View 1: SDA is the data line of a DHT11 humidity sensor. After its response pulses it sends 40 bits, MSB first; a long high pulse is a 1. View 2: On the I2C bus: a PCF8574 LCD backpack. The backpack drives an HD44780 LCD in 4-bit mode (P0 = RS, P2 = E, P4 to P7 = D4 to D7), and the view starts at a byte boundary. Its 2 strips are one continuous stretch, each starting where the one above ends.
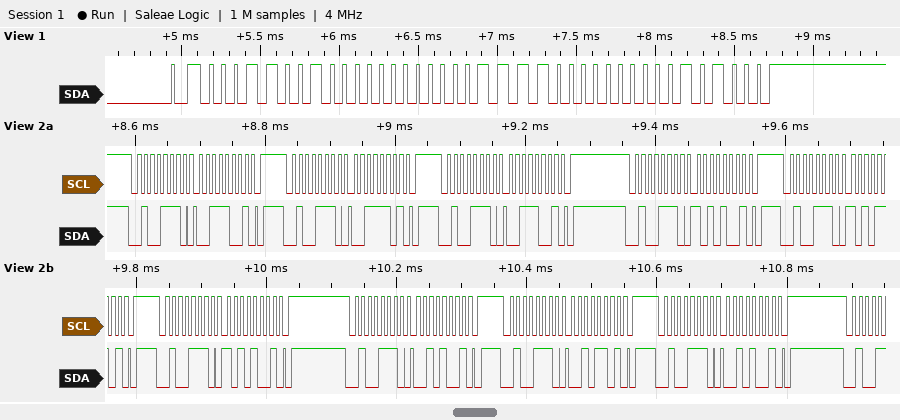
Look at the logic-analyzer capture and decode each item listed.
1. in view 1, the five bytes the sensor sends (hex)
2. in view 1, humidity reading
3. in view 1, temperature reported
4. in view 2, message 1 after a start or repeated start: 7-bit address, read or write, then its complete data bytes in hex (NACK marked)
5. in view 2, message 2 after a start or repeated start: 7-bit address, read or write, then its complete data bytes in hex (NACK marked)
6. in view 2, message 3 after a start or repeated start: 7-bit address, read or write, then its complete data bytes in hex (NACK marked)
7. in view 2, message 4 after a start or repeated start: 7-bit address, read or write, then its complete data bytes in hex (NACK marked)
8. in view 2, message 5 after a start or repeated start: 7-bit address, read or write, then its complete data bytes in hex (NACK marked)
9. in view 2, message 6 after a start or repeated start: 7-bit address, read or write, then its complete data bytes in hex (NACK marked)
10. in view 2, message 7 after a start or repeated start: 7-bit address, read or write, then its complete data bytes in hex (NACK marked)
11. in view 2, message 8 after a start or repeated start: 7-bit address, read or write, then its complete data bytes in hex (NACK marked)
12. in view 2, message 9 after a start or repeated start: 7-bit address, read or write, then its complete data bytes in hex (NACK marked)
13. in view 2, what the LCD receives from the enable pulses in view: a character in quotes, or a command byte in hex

19 00 0F 00 28
25 %
15.0 °C
0x27 write: 39
0x27 write: 3D
0x27 write: 39
0x27 write: A9
0x27 write: AD
0x27 write: A9
0x27 write: 29
0x27 write: 2D
0x27 write: 29
':'
